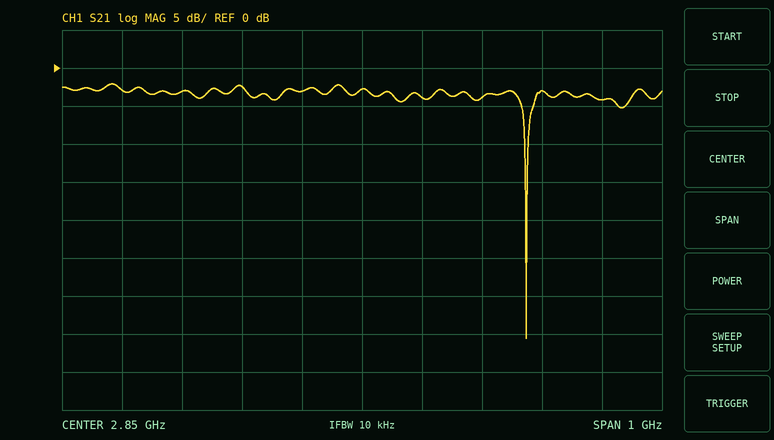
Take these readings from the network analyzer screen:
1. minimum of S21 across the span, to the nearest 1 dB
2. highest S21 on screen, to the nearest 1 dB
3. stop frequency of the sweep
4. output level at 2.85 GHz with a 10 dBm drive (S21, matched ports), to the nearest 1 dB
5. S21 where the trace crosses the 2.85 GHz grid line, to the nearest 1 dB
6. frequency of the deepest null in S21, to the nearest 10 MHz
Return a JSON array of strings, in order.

["-36 dB", "-2 dB", "3.35 GHz", "7 dBm", "-3 dB", "3.12 GHz"]
